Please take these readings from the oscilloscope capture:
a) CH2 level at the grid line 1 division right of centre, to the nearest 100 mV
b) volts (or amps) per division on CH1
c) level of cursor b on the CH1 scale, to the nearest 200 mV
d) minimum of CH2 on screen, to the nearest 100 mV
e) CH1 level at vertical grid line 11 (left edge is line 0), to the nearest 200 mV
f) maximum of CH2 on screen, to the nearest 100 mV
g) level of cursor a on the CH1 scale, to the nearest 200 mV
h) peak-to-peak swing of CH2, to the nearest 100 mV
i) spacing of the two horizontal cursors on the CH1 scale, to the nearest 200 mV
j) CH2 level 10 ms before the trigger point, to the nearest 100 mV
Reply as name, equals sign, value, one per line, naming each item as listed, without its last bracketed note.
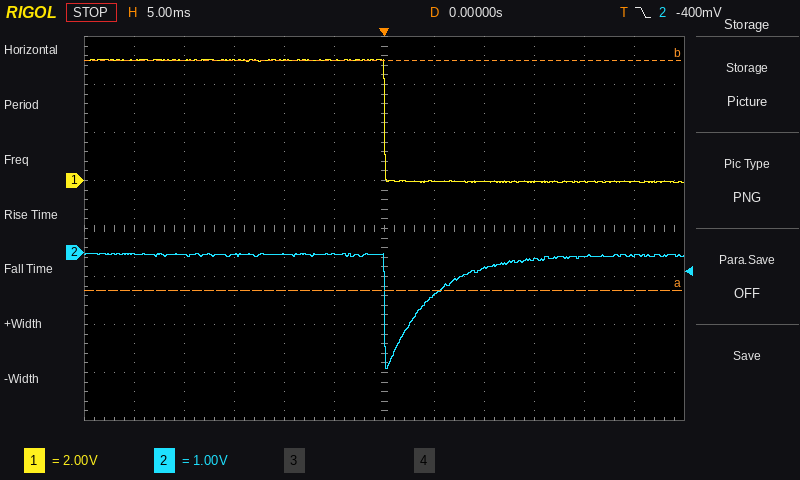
CH2 level at the grid line 1 division right of centre, to the nearest 100 mV = -900 mV
volts (or amps) per division on CH1 = 2 V
level of cursor b on the CH1 scale, to the nearest 200 mV = 5.0 V
minimum of CH2 on screen, to the nearest 100 mV = -2.4 V
CH1 level at vertical grid line 11 (left edge is line 0), to the nearest 200 mV = 0.0 V
maximum of CH2 on screen, to the nearest 100 mV = 0.0 V
level of cursor a on the CH1 scale, to the nearest 200 mV = -4.6 V
peak-to-peak swing of CH2, to the nearest 100 mV = 2.4 V
spacing of the two horizontal cursors on the CH1 scale, to the nearest 200 mV = 9.6 V
CH2 level 10 ms before the trigger point, to the nearest 100 mV = 0.0 V
